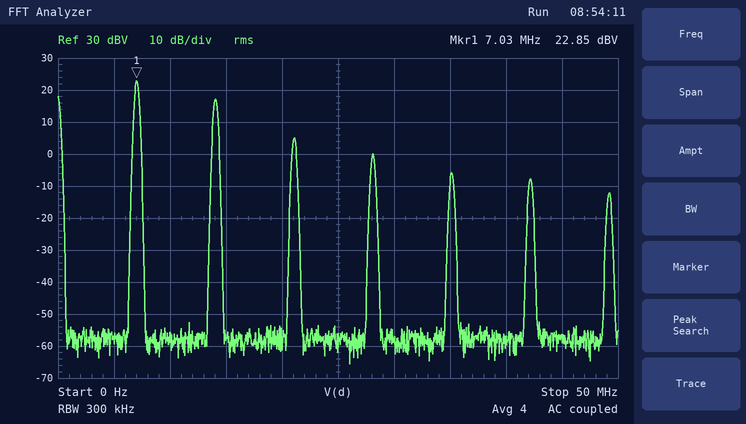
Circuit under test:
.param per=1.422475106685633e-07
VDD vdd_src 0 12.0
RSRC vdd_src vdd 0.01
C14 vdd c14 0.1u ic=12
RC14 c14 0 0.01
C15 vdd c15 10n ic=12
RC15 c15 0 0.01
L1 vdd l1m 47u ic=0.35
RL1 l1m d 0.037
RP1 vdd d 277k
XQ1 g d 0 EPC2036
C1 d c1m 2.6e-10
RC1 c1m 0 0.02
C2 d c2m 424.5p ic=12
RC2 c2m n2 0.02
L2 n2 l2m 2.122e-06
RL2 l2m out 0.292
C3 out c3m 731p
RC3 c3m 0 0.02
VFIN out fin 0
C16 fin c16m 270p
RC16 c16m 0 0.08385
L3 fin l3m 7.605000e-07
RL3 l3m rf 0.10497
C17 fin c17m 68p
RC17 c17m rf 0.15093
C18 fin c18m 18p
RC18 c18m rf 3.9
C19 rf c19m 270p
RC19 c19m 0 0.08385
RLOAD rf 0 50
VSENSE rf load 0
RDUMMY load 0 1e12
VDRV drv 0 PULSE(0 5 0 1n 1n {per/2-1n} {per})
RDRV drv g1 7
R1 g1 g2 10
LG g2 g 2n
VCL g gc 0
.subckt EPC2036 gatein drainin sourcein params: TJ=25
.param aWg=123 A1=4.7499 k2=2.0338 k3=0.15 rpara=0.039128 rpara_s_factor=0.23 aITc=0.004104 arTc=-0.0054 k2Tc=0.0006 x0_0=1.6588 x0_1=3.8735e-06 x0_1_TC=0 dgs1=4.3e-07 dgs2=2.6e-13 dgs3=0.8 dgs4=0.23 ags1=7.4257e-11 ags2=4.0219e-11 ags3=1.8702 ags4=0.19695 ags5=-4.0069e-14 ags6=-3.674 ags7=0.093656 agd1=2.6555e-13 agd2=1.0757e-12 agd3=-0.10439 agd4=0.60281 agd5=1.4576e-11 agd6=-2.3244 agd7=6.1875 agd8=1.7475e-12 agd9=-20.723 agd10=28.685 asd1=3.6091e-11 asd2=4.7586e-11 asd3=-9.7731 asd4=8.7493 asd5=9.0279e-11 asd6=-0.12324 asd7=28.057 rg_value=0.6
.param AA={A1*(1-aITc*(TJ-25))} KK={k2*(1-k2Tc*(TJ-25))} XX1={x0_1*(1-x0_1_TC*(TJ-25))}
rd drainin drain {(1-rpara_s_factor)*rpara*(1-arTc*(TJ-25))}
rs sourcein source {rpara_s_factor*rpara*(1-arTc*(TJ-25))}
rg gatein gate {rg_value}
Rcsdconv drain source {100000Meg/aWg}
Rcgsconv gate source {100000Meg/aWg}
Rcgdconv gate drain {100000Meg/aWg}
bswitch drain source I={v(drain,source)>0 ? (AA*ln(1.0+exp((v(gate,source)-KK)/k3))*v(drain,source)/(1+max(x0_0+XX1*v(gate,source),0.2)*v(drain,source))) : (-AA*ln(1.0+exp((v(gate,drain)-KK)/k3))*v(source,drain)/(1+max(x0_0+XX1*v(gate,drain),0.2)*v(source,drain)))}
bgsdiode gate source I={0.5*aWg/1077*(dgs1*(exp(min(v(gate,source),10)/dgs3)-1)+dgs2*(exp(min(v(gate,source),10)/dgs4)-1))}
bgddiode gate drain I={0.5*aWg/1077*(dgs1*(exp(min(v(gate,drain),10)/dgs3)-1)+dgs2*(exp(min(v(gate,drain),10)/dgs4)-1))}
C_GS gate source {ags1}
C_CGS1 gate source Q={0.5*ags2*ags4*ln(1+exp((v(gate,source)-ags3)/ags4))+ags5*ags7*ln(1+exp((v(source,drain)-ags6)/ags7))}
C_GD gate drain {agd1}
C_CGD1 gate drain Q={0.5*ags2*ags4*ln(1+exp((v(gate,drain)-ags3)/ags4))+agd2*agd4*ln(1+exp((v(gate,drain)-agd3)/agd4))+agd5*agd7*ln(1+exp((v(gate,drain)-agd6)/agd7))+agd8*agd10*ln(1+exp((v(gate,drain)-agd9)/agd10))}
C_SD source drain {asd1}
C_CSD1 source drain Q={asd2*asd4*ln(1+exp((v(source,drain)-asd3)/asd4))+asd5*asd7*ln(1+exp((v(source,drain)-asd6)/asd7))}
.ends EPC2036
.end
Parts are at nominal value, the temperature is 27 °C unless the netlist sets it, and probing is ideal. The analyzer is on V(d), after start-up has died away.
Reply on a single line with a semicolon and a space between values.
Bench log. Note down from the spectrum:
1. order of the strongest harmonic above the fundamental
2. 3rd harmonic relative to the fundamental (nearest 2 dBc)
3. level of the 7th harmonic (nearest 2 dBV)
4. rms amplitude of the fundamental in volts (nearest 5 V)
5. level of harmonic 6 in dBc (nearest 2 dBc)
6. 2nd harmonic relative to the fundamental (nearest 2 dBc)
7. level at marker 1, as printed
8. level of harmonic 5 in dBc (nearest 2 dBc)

2; -18 dBc; -12 dBV; 15 V; -30 dBc; -6 dBc; 22.85 dBV; -28 dBc
